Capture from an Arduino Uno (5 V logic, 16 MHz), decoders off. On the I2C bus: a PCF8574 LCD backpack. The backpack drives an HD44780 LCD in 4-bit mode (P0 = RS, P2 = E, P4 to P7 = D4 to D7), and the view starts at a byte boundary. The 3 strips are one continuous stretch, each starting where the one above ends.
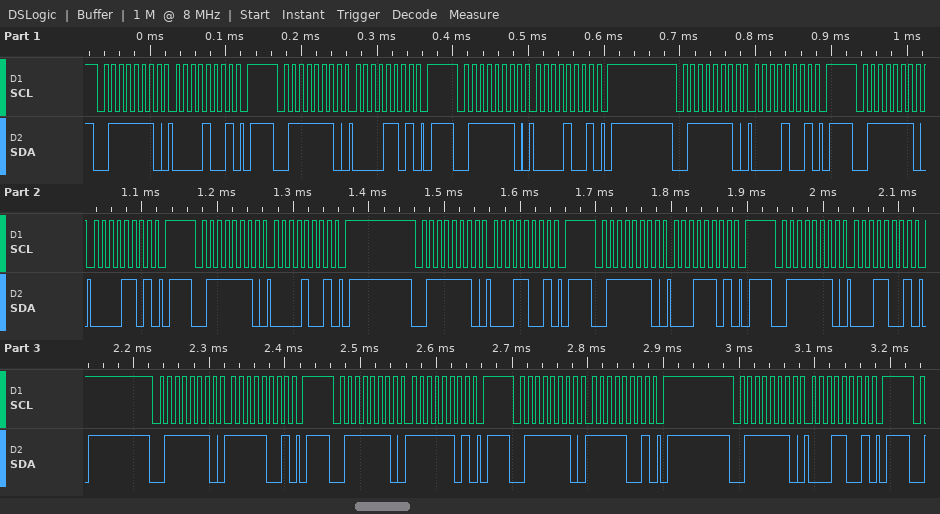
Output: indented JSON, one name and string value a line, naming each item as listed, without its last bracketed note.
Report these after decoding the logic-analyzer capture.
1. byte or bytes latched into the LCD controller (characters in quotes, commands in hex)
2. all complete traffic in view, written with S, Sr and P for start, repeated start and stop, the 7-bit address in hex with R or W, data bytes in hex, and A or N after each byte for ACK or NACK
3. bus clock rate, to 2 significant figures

{
  "byte or bytes latched into the LCD controller": "data 0x00 data 0x1F",
  "all complete traffic in view, written with S, Sr and P for start, repeated start and stop, the 7-bit address in hex with R or W, data bytes in hex, and A or N after each byte for ACK or NACK": "S 3FW A 09 A P S 3FW A 0D A P S 3FW A 09 A P S 3FW A 09 A P S 3FW A 0D A P S 3FW A 09 A P S 3FW A 19 A P S 3FW A 1D A P S 3FW A 19 A P S 3FW A F9 A P S 3FW A FD A P S 3FW A F9 A P S 3FW A 19 A P",
  "bus clock rate, to 2 significant figures": "100 kHz"
}
